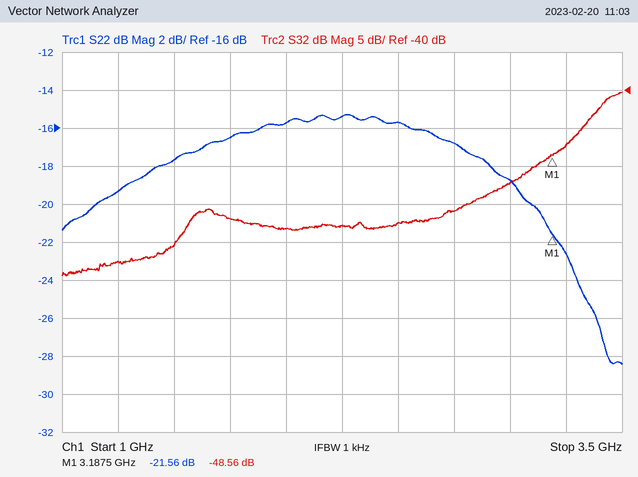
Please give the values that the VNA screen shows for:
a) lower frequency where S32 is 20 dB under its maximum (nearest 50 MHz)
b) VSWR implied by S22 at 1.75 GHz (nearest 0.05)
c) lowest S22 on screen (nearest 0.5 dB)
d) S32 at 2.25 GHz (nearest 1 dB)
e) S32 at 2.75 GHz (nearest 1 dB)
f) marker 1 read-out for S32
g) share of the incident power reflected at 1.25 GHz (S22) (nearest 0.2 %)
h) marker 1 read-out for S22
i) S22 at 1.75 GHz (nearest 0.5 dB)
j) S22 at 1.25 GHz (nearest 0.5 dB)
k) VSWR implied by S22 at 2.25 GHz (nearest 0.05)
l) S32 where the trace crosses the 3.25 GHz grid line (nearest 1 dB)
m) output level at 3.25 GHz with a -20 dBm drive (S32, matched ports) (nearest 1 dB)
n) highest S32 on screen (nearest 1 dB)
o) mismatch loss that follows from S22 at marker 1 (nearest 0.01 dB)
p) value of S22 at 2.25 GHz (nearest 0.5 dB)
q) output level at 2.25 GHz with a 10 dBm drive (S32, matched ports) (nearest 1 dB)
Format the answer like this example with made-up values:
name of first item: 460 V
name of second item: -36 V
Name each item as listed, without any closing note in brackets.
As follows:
lower frequency where S32 is 20 dB under its maximum: 1.50 GHz
VSWR implied by S22 at 1.75 GHz: 1.35
lowest S22 on screen: -28.5 dB
S32 at 2.25 GHz: -58 dB
S32 at 2.75 GHz: -56 dB
marker 1 read-out for S32: -48.56 dB
share of the incident power reflected at 1.25 GHz (S22): 1.2 %
marker 1 read-out for S22: -21.56 dB
S22 at 1.75 GHz: -16.5 dB
S22 at 1.25 GHz: -19.5 dB
VSWR implied by S22 at 2.25 GHz: 1.40
S32 where the trace crosses the 3.25 GHz grid line: -47 dB
output level at 3.25 GHz with a -20 dBm drive (S32, matched ports): -67 dBm
highest S32 on screen: -40 dB
mismatch loss that follows from S22 at marker 1: 0.03 dB
value of S22 at 2.25 GHz: -15.5 dB
output level at 2.25 GHz with a 10 dBm drive (S32, matched ports): -48 dBm
